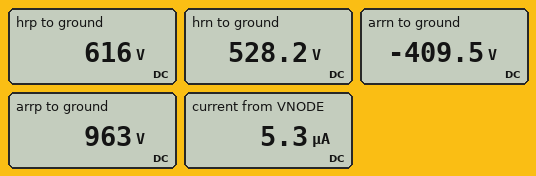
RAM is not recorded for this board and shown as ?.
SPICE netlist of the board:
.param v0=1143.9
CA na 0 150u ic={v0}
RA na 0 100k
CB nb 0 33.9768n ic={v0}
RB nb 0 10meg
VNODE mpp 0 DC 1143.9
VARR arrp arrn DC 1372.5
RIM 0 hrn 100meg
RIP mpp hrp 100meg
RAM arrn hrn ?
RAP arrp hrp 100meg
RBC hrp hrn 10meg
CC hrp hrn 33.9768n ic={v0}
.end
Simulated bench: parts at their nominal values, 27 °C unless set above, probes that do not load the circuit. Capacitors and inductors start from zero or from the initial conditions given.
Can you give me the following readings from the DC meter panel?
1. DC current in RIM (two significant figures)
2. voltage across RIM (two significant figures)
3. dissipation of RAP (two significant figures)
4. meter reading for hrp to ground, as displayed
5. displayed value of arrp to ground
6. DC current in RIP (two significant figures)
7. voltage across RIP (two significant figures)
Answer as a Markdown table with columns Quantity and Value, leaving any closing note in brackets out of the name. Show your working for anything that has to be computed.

| Quantity | Value |
|---|---|
| DC current in RIM | (528.2 V) / 100 MΩ = 5.3 µA |
| voltage across RIM | 528.2 V = 530 V |
| dissipation of RAP | (963 V - 616 V)^2 / 100 MΩ = 1.2 mW |
| meter reading for hrp to ground, as displayed | 616 V |
| displayed value of arrp to ground | 963 V |
| DC current in RIP | (1.144 kV - 616 V) / 100 MΩ = 5.3 µA |
| voltage across RIP | 1.144 kV - 616 V = 530 V |
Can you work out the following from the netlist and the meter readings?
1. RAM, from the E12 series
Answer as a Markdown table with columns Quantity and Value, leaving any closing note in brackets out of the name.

| Quantity | Value |
|---|---|
| RAM, from the E12 series | 270 MΩ |
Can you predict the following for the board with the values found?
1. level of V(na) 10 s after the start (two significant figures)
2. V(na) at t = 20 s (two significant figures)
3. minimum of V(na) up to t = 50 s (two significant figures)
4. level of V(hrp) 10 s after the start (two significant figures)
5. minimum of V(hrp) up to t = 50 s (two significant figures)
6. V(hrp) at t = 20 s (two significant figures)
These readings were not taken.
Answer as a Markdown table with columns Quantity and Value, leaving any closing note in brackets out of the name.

| Quantity | Value |
|---|---|
| level of V(na) 10 s after the start | 590 V |
| V(na) at t = 20 s | 300 V |
| minimum of V(na) up to t = 50 s | 41 V |
| level of V(hrp) 10 s after the start | 620 V |
| minimum of V(hrp) up to t = 50 s | 620 V |
| V(hrp) at t = 20 s | 620 V |
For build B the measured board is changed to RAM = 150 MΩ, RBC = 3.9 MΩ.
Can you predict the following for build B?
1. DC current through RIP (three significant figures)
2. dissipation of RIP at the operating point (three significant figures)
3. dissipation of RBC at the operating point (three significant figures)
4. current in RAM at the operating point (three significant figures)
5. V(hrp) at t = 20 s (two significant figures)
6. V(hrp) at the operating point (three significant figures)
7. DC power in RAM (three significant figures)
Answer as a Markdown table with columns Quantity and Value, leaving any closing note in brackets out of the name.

| Quantity | Value |
|---|---|
| DC current through RIP | 5.51 µA |
| dissipation of RIP at the operating point | 3.03 mW |
| dissipation of RBC at the operating point | 457 µW |
| current in RAM at the operating point | 5.32 µA |
| V(hrp) at t = 20 s | 590 V |
| V(hrp) at the operating point | 593 V |
| DC power in RAM | 4.25 mW |
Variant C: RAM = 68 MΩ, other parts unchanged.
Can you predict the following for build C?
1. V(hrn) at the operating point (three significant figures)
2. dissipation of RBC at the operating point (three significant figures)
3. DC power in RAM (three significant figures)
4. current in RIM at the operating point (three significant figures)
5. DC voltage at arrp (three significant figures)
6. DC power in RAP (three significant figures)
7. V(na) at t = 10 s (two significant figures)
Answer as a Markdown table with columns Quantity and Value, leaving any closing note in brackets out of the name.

| Quantity | Value |
|---|---|
| V(hrn) at the operating point | 509 V |
| dissipation of RBC at the operating point | 1.57 mW |
| DC power in RAM | 3.75 mW |
| current in RIM at the operating point | 5.09 µA |
| DC voltage at arrp | 1.38 kV |
| DC power in RAP | 5.51 mW |
| V(na) at t = 10 s | 590 V |
